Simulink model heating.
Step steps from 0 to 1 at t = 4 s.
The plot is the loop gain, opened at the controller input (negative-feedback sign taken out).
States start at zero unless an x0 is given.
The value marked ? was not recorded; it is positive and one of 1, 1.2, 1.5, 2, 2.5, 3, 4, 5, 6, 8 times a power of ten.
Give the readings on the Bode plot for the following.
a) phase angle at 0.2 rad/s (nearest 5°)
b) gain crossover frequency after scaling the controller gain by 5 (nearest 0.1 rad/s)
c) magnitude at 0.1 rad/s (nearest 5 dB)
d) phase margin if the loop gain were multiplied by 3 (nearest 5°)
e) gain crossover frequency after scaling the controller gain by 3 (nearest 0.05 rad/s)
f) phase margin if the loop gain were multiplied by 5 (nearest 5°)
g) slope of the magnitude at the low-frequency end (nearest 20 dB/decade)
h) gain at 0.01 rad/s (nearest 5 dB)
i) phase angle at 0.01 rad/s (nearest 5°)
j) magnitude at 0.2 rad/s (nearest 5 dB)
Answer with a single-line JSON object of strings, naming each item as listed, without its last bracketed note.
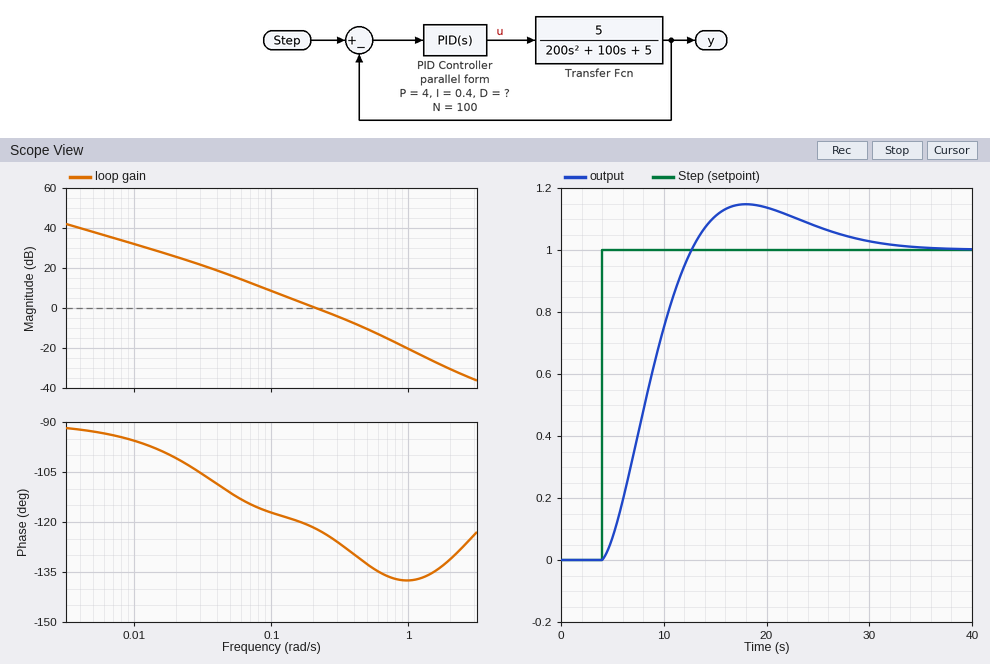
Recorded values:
{"phase angle at 0.2 rad/s": "-120°", "gain crossover frequency after scaling the controller gain by 5": "0.6 rad/s", "magnitude at 0.1 rad/s": "10 dB", "phase margin if the loop gain were multiplied by 3": "50°", "gain crossover frequency after scaling the controller gain by 3": "0.45 rad/s", "phase margin if the loop gain were multiplied by 5": "45°", "slope of the magnitude at the low-frequency end": "-20 dB/decade", "gain at 0.01 rad/s": "30 dB", "phase angle at 0.01 rad/s": "-95°", "magnitude at 0.2 rad/s": "0 dB"}
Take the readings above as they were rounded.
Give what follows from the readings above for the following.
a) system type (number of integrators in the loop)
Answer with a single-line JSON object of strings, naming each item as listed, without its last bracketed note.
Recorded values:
{"system type": "1"}
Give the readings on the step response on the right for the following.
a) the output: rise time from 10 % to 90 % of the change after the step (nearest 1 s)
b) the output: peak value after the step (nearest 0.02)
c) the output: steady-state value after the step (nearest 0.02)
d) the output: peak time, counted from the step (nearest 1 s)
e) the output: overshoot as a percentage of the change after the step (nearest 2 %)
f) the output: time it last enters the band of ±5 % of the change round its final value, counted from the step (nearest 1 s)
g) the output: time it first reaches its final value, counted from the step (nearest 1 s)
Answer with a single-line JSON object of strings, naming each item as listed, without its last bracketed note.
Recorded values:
{"the output: rise time from 10 % to 90 % of the change after the step": "6 s", "the output: peak value after the step": "1.14", "the output: steady-state value after the step": "1.00", "the output: peak time, counted from the step": "14 s", "the output: overshoot as a percentage of the change after the step": "14 %", "the output: time it last enters the band of ±5 % of the change round its final value, counted from the step": "23 s", "the output: time it first reaches its final value, counted from the step": "9 s"}
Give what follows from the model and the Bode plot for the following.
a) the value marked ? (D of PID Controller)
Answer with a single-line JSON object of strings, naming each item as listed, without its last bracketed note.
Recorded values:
{"the value marked ?": "1.5"}
